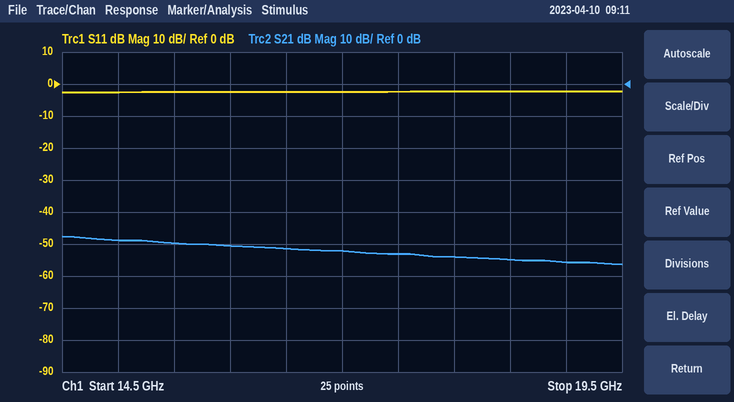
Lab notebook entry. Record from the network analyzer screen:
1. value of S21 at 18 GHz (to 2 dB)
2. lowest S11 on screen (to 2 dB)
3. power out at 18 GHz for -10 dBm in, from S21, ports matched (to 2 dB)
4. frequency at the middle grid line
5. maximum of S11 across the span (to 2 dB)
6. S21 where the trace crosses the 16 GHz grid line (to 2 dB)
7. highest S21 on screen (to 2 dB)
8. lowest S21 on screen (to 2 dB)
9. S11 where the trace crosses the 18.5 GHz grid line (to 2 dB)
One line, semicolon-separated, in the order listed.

-54 dB; -2 dB; -64 dBm; 17 GHz; -2 dB; -50 dB; -48 dB; -56 dB; -2 dB
